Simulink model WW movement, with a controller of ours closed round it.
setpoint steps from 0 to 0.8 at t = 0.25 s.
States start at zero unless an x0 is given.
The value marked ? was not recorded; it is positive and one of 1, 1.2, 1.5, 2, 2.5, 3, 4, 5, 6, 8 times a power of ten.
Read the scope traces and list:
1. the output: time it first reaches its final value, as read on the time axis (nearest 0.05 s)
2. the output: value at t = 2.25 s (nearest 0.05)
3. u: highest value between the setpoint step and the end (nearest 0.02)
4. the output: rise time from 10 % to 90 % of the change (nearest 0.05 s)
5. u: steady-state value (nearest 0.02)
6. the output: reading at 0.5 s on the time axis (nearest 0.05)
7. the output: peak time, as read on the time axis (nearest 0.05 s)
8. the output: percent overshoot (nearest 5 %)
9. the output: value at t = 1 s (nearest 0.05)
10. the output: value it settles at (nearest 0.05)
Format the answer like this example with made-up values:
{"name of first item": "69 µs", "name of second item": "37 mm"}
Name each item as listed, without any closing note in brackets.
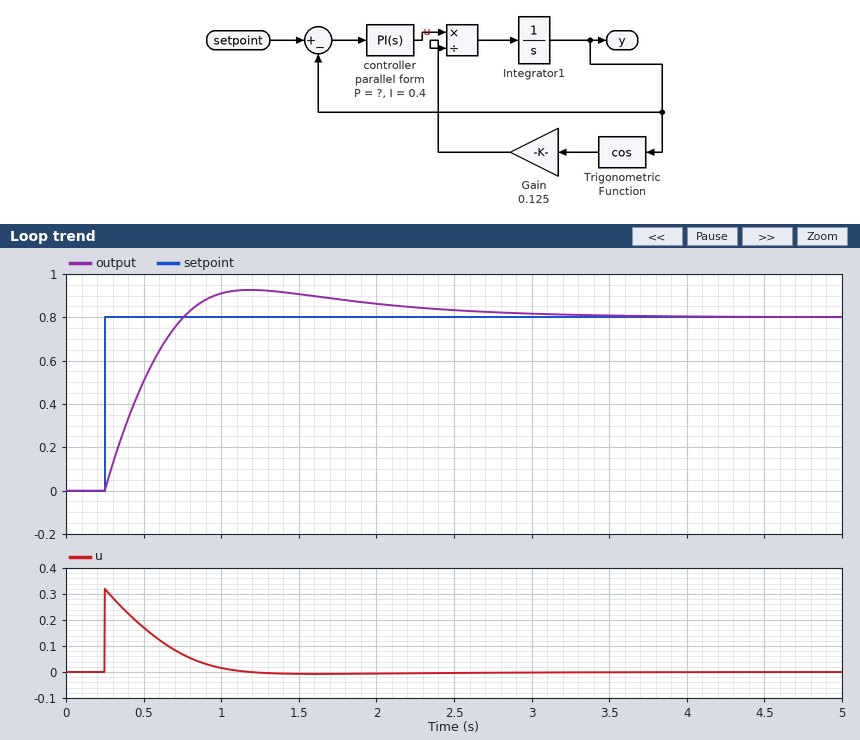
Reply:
{"the output: time it first reaches its final value, as read on the time axis": "0.75 s", "the output: value at t = 2.25 s": "0.85", "u: highest value between the setpoint step and the end": "0.32", "the output: rise time from 10 % to 90 % of the change": "0.40 s", "u: steady-state value": "0.00", "the output: reading at 0.5 s on the time axis": "0.50", "the output: peak time, as read on the time axis": "1.20 s", "the output: percent overshoot": "15 %", "the output: value at t = 1 s": "0.90", "the output: value it settles at": "0.80"}
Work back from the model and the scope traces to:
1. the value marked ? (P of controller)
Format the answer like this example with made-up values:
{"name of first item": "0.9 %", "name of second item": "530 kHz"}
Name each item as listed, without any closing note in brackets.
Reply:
{"the value marked ?": "0.4"}
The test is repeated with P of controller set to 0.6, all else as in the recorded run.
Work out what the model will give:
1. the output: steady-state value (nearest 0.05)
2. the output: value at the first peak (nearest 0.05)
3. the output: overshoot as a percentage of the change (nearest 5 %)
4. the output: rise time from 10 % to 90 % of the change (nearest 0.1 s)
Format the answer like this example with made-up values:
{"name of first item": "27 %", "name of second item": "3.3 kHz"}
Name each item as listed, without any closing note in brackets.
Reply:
{"the output: steady-state value": "0.80", "the output: value at the first peak": "0.85", "the output: overshoot as a percentage of the change": "10 %", "the output: rise time from 10 % to 90 % of the change": "0.3 s"}
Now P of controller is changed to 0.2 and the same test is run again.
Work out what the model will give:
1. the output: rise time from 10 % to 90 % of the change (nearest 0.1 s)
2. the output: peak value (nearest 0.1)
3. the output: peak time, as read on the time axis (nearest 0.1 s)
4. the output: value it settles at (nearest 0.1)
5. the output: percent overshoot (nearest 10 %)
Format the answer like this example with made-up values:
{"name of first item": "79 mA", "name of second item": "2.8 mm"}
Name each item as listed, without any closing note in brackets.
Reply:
{"the output: rise time from 10 % to 90 % of the change": "0.5 s", "the output: peak value": "1.1", "the output: peak time, as read on the time axis": "1.4 s", "the output: value it settles at": "0.8", "the output: percent overshoot": "40 %"}
